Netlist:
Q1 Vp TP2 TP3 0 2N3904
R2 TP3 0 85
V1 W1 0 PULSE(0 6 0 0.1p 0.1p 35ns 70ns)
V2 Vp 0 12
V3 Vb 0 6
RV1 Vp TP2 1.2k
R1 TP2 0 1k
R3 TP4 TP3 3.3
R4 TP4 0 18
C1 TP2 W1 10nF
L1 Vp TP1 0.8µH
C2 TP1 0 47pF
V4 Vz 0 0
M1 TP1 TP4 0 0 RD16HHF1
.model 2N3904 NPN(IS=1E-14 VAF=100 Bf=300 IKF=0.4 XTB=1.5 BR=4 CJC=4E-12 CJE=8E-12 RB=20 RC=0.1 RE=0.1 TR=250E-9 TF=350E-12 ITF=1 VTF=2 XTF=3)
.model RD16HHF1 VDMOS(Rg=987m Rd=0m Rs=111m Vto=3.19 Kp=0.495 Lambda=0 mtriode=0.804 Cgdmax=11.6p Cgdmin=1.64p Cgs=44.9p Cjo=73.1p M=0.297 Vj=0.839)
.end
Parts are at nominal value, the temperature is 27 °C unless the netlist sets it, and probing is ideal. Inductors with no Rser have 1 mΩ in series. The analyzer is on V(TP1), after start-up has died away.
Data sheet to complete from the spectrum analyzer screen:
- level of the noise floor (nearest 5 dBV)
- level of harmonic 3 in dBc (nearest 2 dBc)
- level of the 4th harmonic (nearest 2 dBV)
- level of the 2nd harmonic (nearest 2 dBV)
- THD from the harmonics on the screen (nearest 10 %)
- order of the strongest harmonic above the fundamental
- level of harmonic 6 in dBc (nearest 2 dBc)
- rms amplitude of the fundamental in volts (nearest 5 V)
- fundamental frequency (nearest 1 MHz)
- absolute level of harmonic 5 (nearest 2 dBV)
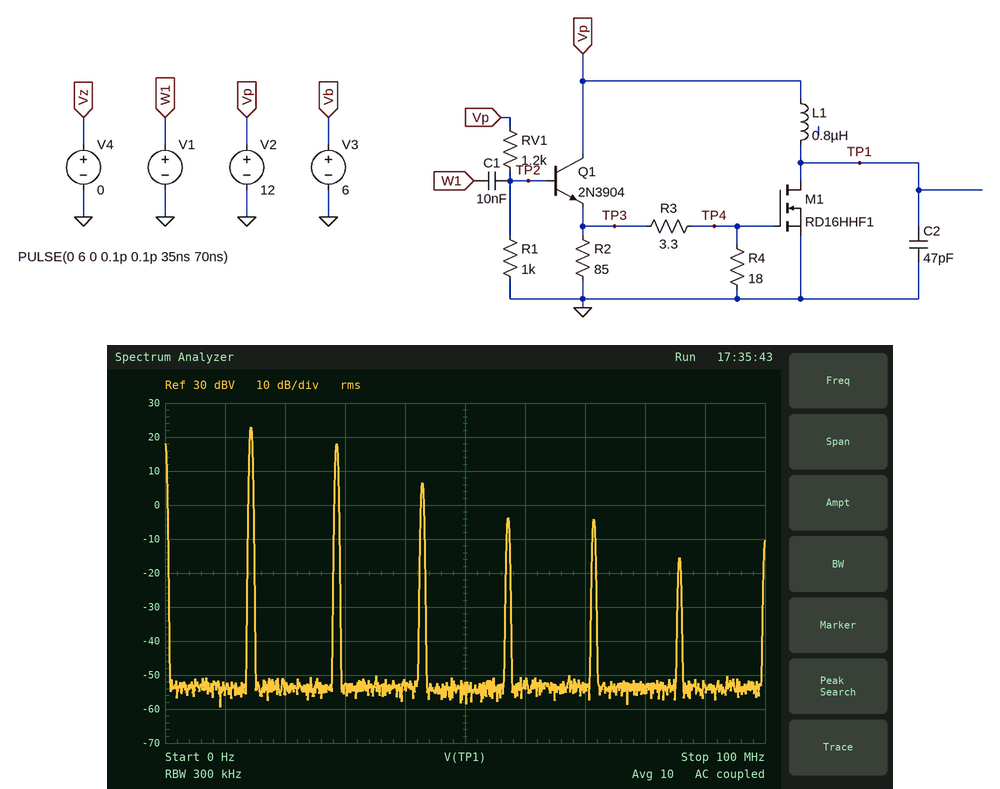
-55 dBV
-16 dBc
-4 dBV
18 dBV
60 %
2
-38 dBc
15 V
14 MHz
-4 dBV
